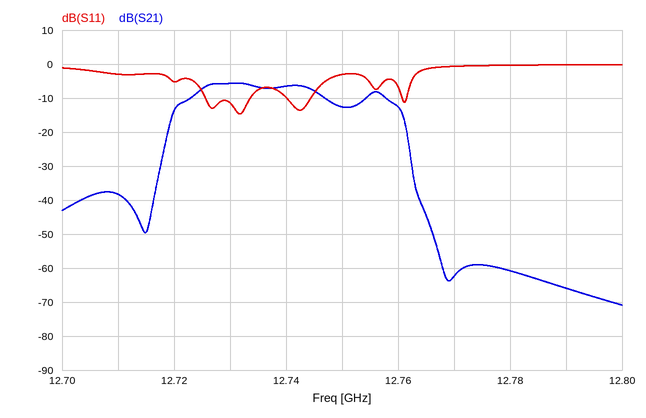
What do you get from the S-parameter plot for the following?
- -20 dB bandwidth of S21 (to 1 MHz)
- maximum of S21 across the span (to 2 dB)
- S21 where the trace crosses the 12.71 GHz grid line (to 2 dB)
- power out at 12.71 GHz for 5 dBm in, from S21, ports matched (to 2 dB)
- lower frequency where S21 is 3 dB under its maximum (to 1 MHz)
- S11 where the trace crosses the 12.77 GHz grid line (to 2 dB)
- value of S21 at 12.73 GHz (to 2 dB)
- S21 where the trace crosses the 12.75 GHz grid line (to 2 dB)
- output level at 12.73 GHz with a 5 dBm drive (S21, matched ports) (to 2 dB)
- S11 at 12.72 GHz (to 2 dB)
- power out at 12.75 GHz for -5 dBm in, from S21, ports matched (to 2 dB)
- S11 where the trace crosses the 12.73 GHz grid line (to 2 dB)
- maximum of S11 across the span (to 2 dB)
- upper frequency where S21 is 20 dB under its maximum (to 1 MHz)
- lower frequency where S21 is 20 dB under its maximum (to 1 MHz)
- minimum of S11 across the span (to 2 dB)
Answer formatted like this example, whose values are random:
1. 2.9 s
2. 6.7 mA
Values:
1. 44 MHz
2. -6 dB
3. -38 dB
4. -34 dBm
5. 12.724 GHz
6. 0 dB
7. -6 dB
8. -12 dB
9. 0 dBm
10. -6 dB
11. -18 dBm
12. -12 dB
13. 0 dB
14. 12.762 GHz
15. 12.718 GHz
16. -14 dB
